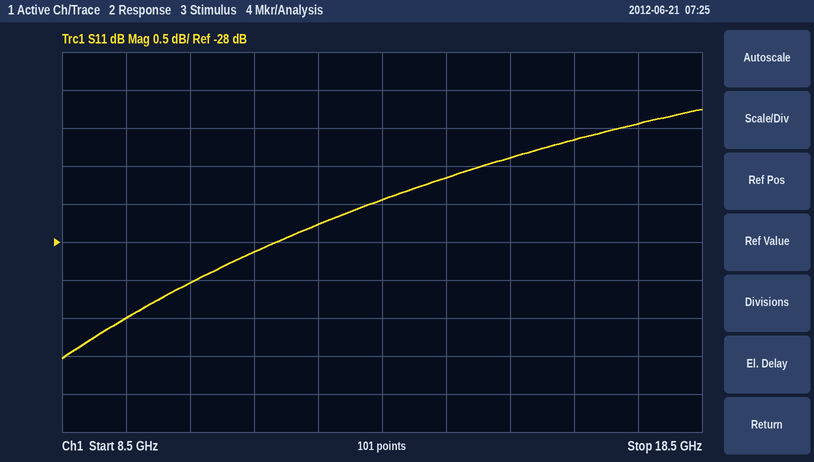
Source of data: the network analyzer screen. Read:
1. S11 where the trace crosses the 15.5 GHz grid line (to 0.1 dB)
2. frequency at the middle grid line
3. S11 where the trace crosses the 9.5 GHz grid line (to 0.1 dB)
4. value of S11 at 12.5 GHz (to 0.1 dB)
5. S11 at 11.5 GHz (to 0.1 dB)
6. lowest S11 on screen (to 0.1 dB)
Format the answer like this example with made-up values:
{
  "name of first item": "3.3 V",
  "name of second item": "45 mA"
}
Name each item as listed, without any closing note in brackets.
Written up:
{
  "S11 where the trace crosses the 15.5 GHz grid line": "-26.9 dB",
  "frequency at the middle grid line": "13.5 GHz",
  "S11 where the trace crosses the 9.5 GHz grid line": "-29.0 dB",
  "value of S11 at 12.5 GHz": "-27.8 dB",
  "S11 at 11.5 GHz": "-28.1 dB",
  "lowest S11 on screen": "-29.5 dB"
}
